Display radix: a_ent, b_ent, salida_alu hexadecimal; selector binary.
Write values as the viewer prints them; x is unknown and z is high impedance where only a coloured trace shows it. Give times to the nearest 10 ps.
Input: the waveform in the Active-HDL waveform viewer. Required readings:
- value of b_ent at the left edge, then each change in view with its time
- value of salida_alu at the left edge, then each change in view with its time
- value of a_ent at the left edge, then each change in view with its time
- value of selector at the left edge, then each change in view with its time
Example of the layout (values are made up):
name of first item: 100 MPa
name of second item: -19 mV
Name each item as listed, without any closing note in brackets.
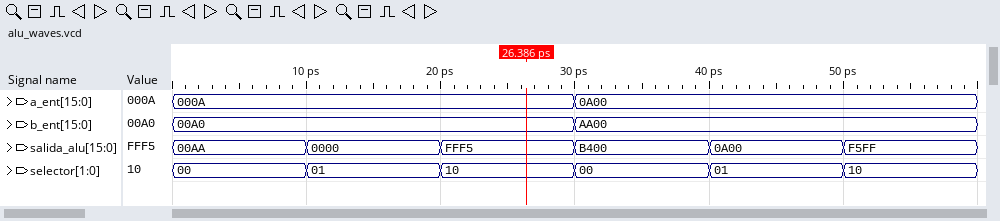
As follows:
value of b_ent at the left edge, then each change in view with its time: 00A0, AA00 at 30 ps
value of salida_alu at the left edge, then each change in view with its time: 00AA, 0000 at 10 ps, FFF5 at 20 ps, B400 at 30 ps, 0A00 at 40 ps, F5FF at 50 ps
value of a_ent at the left edge, then each change in view with its time: 000A, 0A00 at 30 ps
value of selector at the left edge, then each change in view with its time: 00, 01 at 10 ps, 10 at 20 ps, 00 at 30 ps, 01 at 40 ps, 10 at 50 ps
